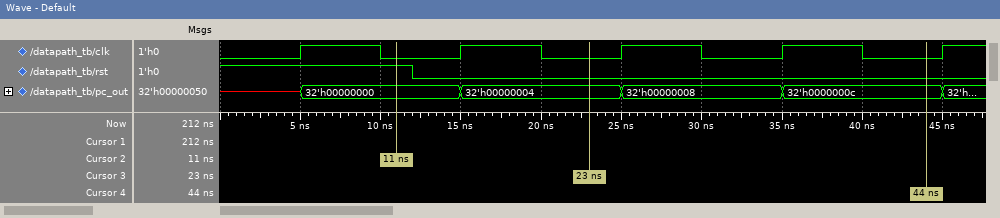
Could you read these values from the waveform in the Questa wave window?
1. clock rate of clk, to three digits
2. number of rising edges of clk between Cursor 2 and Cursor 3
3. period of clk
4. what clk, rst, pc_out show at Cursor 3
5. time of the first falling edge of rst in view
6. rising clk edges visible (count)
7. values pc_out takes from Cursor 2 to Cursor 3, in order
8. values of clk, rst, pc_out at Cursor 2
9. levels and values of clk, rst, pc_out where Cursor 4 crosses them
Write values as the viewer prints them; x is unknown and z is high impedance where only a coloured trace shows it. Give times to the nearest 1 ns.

100 MHz
1
10 ns
clk=0, rst=0, pc_out=32'h00000004
12 ns
5
32'h00000000, 32'h00000004
clk=0, rst=1, pc_out=32'h00000000
clk=0, rst=0, pc_out=32'h0000000c
